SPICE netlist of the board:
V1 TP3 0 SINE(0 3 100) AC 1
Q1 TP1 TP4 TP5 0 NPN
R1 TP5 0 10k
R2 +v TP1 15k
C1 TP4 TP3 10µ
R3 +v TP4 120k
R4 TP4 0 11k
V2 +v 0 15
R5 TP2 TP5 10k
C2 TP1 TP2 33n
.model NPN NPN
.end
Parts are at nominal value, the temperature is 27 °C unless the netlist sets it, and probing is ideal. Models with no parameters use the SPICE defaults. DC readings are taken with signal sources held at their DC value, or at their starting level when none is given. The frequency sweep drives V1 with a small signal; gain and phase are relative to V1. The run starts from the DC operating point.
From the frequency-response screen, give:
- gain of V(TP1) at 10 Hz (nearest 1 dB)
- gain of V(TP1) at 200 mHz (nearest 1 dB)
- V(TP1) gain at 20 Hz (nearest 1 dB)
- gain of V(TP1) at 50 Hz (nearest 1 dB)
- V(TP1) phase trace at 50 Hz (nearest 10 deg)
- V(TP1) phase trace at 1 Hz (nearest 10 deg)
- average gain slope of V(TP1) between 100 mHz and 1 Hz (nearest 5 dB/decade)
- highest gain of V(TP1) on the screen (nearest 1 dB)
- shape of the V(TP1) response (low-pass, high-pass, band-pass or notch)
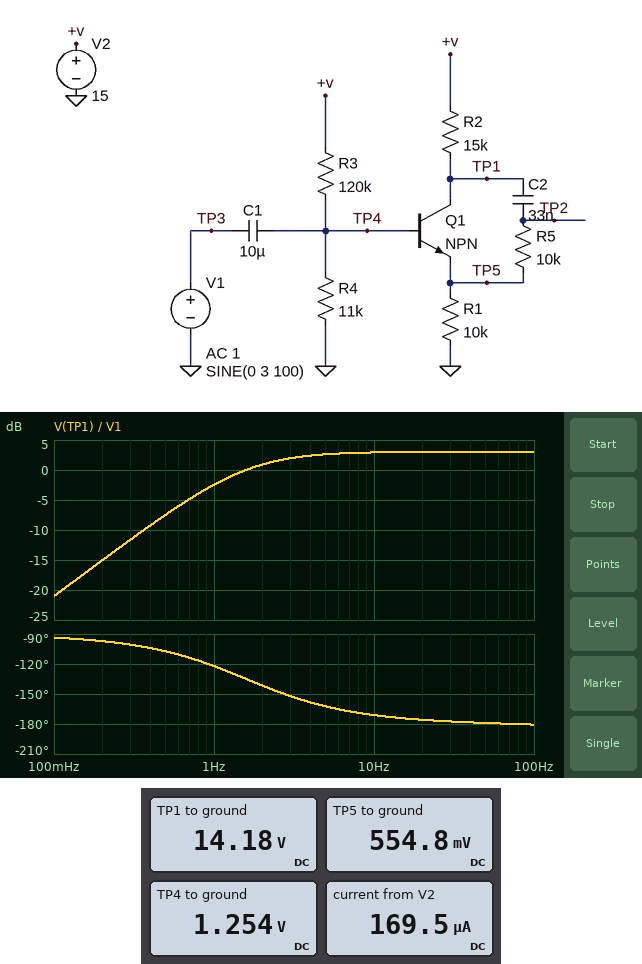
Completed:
3 dB
-15 dB
3 dB
3 dB
-180 deg
-120 deg
20 dB/decade
3 dB
high-pass
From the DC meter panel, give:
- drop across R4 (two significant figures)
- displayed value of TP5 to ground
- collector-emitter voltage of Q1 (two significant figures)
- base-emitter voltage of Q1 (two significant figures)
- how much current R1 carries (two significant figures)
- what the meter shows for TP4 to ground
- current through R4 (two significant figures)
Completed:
1.3 V
554.8 mV
14 V
700 mV
55 µA
1.254 V
110 µA
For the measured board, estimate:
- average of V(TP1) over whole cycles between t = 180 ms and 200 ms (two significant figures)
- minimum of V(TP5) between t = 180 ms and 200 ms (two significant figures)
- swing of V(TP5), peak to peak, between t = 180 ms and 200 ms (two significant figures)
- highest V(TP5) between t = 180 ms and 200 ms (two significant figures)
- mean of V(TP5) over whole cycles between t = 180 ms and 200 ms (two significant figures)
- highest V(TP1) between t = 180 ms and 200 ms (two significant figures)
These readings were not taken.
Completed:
13 V
17 mV
3.5 V
3.5 V
1.3 V
15 V
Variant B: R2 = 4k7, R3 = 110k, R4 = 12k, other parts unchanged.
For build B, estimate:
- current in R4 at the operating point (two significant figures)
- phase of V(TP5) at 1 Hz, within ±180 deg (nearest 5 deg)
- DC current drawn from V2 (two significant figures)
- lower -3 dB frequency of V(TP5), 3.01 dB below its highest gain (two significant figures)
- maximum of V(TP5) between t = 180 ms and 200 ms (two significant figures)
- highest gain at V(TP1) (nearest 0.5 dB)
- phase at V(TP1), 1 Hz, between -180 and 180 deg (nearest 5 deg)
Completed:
120 µA
55 deg
200 µA
1.5 Hz
3.7 V
-7.0 dB
-125 deg
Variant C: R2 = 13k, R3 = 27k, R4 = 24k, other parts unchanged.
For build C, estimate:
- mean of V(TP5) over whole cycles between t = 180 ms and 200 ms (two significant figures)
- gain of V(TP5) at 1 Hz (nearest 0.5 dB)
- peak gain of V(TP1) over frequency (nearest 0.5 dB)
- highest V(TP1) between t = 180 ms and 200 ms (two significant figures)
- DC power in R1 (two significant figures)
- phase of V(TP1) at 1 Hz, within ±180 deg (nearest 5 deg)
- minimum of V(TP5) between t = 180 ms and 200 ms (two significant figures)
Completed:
5.4 V
-4.0 dB
2.0 dB
12 V
3.9 mW
-130 deg
2.4 V
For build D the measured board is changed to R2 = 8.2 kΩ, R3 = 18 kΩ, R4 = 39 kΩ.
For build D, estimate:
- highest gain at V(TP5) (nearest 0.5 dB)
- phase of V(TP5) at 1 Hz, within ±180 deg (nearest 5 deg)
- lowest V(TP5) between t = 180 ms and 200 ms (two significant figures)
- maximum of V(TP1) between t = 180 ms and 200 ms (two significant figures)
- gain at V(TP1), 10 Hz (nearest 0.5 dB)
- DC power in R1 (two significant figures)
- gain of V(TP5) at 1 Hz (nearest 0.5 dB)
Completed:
0 dB
80 deg
4.7 V
11 V
-1.5 dB
7.3 mW
-13.5 dB
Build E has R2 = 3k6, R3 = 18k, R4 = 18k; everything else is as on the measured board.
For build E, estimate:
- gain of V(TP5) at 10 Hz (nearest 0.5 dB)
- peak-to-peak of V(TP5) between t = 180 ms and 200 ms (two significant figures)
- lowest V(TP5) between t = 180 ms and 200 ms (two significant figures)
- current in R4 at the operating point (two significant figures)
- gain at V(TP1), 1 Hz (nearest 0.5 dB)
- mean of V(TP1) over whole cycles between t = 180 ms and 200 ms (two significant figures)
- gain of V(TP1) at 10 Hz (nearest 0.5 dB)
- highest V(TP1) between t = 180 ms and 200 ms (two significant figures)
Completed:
0 dB
6.0 V
3.7 V
410 µA
-15.0 dB
13 V
-9.0 dB
14 V
